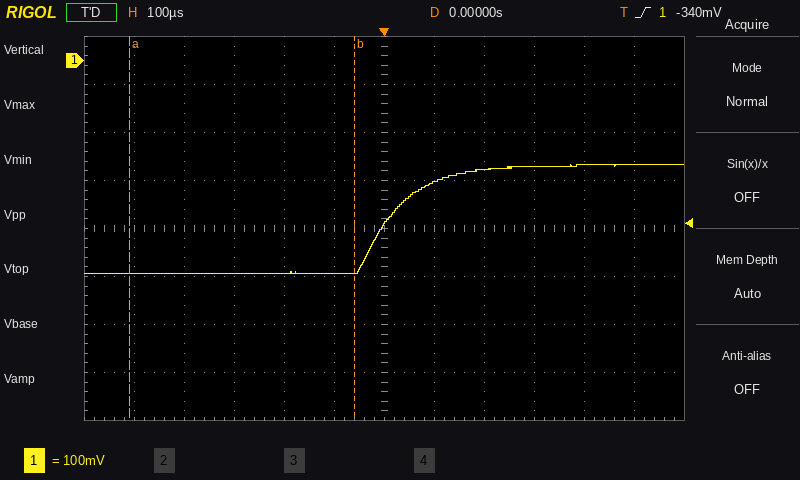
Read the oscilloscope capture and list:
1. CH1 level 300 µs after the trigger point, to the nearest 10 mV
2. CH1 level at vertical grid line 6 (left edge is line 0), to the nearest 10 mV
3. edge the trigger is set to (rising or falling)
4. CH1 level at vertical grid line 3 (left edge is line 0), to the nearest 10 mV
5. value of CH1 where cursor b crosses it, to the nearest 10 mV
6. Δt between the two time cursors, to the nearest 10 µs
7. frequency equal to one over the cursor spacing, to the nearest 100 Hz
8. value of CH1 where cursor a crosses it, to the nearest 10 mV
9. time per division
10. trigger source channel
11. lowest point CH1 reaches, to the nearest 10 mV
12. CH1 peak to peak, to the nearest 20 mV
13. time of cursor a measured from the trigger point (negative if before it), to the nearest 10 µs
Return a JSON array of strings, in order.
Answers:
["-220 mV", "-340 mV", "rising", "-440 mV", "-440 mV", "450 µs", "2.2 kHz", "-440 mV", "100 µs", "CH1", "-440 mV", "220 mV", "-510 µs"]
